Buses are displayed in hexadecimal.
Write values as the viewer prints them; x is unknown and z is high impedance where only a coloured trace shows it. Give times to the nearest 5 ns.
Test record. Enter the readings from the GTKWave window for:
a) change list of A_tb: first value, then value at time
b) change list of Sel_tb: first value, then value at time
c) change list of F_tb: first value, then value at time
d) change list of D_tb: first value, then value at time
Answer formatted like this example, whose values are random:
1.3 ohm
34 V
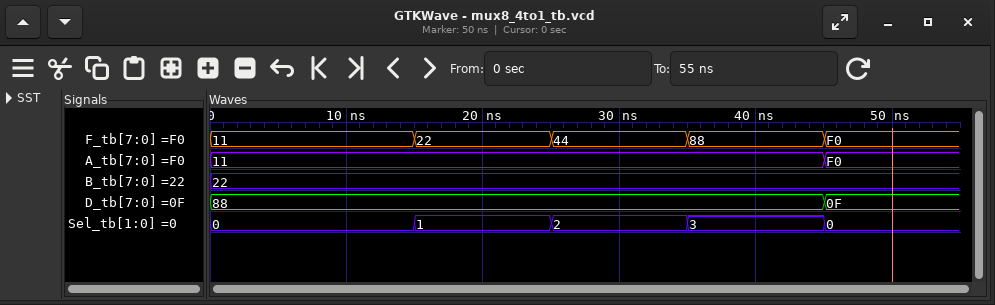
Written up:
11, F0 at 45 ns
0, 1 at 15 ns, 2 at 25 ns, 3 at 35 ns, 0 at 45 ns
11, 22 at 15 ns, 44 at 25 ns, 88 at 35 ns, F0 at 45 ns
88, 0F at 45 ns
